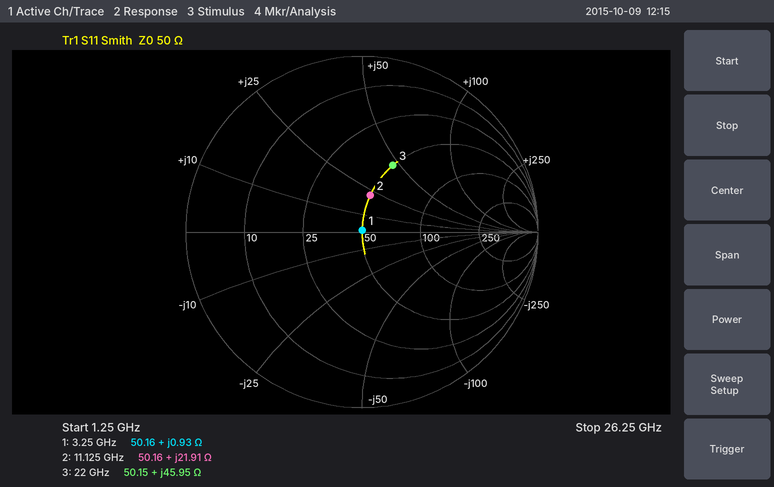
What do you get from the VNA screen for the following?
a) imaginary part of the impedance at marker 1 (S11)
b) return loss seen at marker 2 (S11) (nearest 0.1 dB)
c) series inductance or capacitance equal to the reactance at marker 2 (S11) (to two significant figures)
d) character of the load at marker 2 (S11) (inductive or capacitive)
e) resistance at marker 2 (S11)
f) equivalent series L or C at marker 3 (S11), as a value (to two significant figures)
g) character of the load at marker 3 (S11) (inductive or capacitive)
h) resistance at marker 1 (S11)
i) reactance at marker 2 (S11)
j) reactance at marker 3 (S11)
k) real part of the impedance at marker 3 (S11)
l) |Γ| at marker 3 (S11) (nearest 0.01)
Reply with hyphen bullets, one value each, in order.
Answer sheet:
- +0.93 Ω
- 13.4 dB
- 310 pH
- inductive
- 50.16 Ω
- 330 pH
- inductive
- 50.16 Ω
- +21.91 Ω
- +45.95 Ω
- 50.15 Ω
- 0.42
